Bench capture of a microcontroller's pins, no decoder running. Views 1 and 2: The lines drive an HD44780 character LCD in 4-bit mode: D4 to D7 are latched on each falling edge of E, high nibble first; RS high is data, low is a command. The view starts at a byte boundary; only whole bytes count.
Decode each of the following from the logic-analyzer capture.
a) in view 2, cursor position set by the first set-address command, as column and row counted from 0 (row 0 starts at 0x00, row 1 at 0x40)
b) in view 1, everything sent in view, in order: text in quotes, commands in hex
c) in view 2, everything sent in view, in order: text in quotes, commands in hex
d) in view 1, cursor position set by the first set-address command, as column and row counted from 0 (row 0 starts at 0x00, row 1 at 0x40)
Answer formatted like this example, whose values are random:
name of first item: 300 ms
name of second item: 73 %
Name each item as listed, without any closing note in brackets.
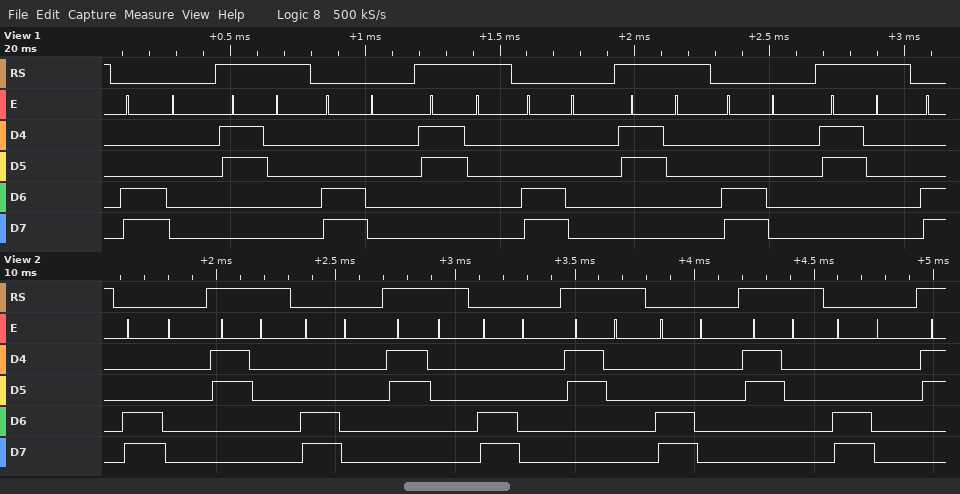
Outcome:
in view 2, cursor position set by the first set-address command, as column and row counted from 0: column 0, row 1
in view 1, everything sent in view, in order: text in quotes, commands in hex: 0xC0 "0" 0xC0 "0" 0xC0 "0" 0xC0 "0"
in view 2, everything sent in view, in order: text in quotes, commands in hex: 0xC0 "0" 0xC0 "0" 0xC0 "0" 0xC0 "0" 0xC0
in view 1, cursor position set by the first set-address command, as column and row counted from 0: column 0, row 1
